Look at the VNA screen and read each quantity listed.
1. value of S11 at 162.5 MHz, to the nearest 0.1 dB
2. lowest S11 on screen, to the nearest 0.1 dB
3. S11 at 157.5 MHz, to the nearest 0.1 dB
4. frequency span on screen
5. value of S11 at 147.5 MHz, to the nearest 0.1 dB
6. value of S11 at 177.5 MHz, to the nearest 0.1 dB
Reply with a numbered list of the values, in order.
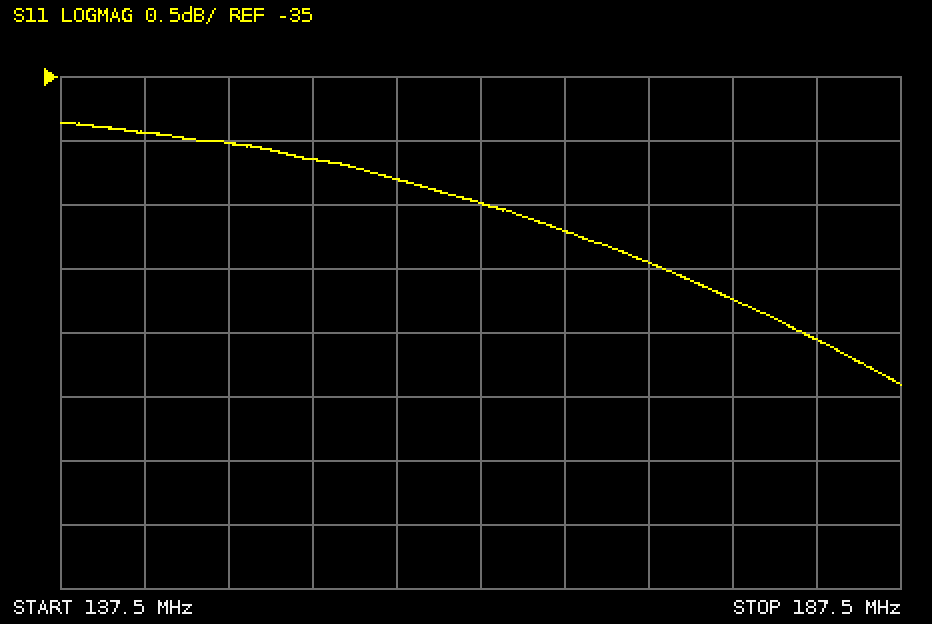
1. -36.0 dB
2. -37.4 dB
3. -35.8 dB
4. 50 MHz
5. -35.5 dB
6. -36.7 dB
